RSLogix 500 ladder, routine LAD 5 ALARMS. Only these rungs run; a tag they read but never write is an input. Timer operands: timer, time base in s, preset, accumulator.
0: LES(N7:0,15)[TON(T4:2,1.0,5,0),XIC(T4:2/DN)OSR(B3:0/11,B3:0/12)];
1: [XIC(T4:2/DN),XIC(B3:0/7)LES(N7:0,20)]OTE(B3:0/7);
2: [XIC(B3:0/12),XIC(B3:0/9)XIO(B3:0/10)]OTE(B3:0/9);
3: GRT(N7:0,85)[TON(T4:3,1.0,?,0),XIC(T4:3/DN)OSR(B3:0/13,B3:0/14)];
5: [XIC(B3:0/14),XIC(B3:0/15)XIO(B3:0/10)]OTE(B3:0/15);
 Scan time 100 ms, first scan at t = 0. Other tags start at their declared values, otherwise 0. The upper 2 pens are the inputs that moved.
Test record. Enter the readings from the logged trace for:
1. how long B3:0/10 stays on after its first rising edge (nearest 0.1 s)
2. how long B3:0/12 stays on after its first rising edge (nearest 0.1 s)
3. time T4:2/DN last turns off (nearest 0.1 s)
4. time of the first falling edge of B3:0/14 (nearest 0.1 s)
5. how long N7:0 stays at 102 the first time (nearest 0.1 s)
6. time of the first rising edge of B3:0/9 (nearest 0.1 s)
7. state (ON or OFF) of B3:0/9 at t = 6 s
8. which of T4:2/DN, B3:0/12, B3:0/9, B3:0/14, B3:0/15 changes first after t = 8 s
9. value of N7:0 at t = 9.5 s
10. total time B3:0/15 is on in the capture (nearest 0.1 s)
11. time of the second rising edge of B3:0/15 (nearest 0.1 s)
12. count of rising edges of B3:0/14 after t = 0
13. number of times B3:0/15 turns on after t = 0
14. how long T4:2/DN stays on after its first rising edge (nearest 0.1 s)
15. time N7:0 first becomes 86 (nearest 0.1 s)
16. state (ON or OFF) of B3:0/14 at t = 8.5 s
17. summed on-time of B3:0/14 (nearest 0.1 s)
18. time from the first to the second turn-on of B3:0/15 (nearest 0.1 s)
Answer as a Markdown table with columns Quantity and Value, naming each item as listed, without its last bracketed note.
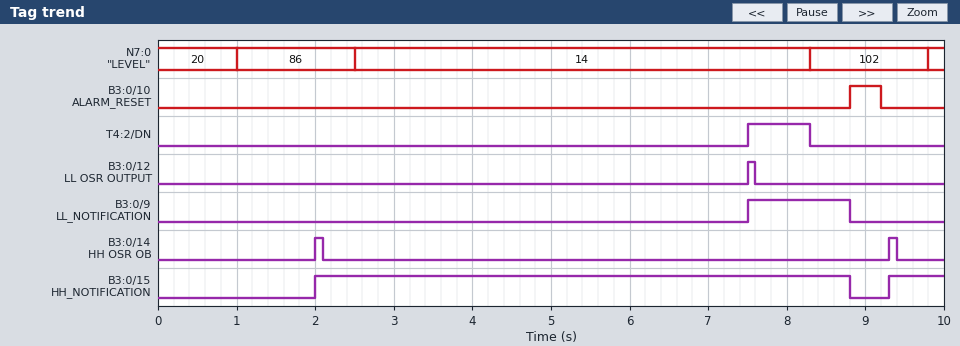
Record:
| Quantity | Value |
|---|---|
| how long B3:0/10 stays on after its first rising edge | 0.4 s |
| how long B3:0/12 stays on after its first rising edge | 0.1 s |
| time T4:2/DN last turns off | 8.3 s |
| time of the first falling edge of B3:0/14 | 2.1 s |
| how long N7:0 stays at 102 the first time | 1.5 s |
| time of the first rising edge of B3:0/9 | 7.5 s |
| state (ON or OFF) of B3:0/9 at t = 6 s | OFF |
| which of T4:2/DN, B3:0/12, B3:0/9, B3:0/14, B3:0/15 changes first after t = 8 s | T4:2/DN |
| value of N7:0 at t = 9.5 s | 102 |
| total time B3:0/15 is on in the capture | 7.5 s |
| time of the second rising edge of B3:0/15 | 9.3 s |
| count of rising edges of B3:0/14 after t = 0 | 2 |
| number of times B3:0/15 turns on after t = 0 | 2 |
| how long T4:2/DN stays on after its first rising edge | 0.8 s |
| time N7:0 first becomes 86 | 1.0 s |
| state (ON or OFF) of B3:0/14 at t = 8.5 s | OFF |
| summed on-time of B3:0/14 | 0.2 s |
| time from the first to the second turn-on of B3:0/15 | 7.3 s |
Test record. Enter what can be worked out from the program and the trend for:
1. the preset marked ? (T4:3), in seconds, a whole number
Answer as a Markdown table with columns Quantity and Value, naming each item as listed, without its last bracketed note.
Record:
| Quantity | Value |
|---|---|
| the preset marked ? (T4:3), in seconds, a whole number | 1 s |
